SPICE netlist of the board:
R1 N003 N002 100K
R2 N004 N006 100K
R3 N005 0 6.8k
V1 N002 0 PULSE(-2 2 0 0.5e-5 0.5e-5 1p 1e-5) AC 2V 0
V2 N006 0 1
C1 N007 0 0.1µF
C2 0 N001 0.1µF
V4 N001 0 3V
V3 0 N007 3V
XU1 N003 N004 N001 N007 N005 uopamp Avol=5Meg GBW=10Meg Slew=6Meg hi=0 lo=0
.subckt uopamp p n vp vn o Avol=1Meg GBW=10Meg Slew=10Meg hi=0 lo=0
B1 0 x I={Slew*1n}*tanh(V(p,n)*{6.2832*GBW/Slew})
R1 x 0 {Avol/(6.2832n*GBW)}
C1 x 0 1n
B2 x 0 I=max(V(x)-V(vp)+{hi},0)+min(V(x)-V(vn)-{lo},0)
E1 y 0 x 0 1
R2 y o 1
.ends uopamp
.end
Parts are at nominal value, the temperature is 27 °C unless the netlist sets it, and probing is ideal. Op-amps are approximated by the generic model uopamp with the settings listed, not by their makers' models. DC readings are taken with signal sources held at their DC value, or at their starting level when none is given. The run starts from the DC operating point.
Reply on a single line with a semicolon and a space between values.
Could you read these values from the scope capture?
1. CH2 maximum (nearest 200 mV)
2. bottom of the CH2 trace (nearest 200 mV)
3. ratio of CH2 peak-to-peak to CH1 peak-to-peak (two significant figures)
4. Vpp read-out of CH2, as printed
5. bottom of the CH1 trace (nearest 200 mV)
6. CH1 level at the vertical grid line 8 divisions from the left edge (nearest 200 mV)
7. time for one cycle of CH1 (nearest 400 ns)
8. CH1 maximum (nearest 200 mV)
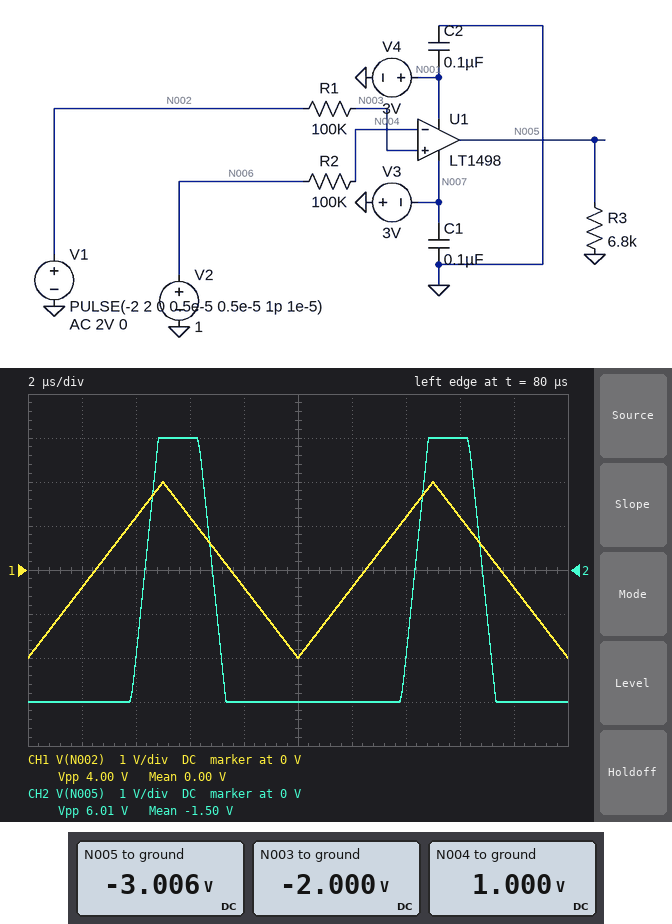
3.0 V; -3.0 V; 1.5; 6.01 V; -2.0 V; 1.2 V; 10.0 µs; 2.0 V
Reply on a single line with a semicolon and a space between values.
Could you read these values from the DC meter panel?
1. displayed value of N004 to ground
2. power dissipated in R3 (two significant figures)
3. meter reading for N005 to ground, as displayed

1.000 V; 1.3 mW; -3.006 V
